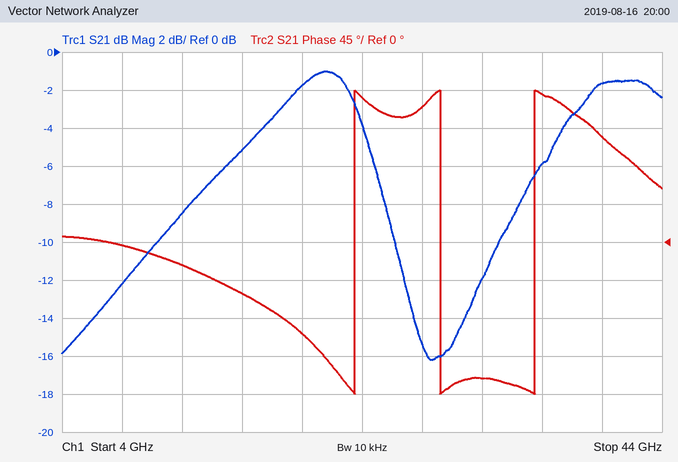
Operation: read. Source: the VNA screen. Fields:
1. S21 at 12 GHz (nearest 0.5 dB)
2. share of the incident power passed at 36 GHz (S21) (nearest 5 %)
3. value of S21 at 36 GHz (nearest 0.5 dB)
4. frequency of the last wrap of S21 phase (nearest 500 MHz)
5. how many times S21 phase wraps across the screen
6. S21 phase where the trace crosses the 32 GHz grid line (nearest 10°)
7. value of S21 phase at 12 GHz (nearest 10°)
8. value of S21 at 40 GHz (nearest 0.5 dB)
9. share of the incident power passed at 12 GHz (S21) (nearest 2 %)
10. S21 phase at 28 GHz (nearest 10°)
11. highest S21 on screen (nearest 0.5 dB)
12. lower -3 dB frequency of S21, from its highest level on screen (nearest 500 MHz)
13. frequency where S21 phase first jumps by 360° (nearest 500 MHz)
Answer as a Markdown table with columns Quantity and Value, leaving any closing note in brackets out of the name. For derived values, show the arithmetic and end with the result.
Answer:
| Quantity | Value |
|---|---|
| S21 at 12 GHz | -8.5 dB |
| share of the incident power passed at 36 GHz (S21) | 10^(-6/10) ≈ 25 % |
| value of S21 at 36 GHz | -6.0 dB |
| frequency of the last wrap of S21 phase | 35.5 GHz |
| how many times S21 phase wraps across the screen | 3 |
| S21 phase where the trace crosses the 32 GHz grid line | -160° |
| value of S21 phase at 12 GHz | -30° |
| value of S21 at 40 GHz | -1.5 dB |
| share of the incident power passed at 12 GHz (S21) | 10^(-8.5/10) ≈ 14 % |
| S21 phase at 28 GHz | 160° |
| highest S21 on screen | -1.0 dB |
| lower -3 dB frequency of S21, from its highest level on screen | 17.5 GHz |
| frequency where S21 phase first jumps by 360° | 23.5 GHz |
